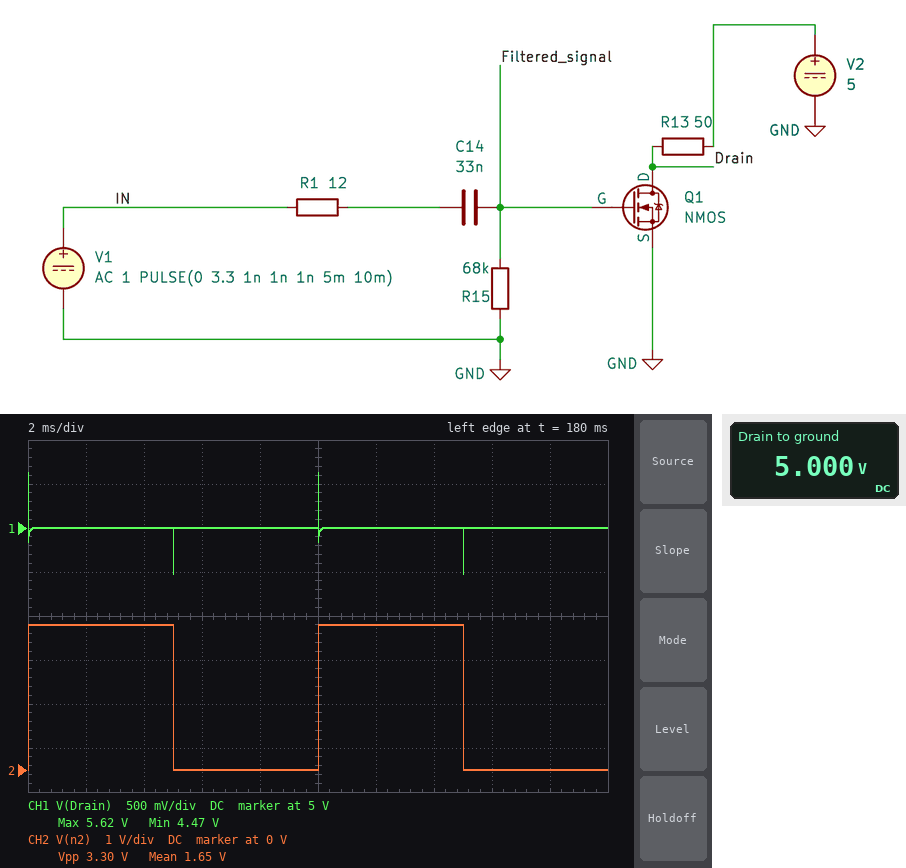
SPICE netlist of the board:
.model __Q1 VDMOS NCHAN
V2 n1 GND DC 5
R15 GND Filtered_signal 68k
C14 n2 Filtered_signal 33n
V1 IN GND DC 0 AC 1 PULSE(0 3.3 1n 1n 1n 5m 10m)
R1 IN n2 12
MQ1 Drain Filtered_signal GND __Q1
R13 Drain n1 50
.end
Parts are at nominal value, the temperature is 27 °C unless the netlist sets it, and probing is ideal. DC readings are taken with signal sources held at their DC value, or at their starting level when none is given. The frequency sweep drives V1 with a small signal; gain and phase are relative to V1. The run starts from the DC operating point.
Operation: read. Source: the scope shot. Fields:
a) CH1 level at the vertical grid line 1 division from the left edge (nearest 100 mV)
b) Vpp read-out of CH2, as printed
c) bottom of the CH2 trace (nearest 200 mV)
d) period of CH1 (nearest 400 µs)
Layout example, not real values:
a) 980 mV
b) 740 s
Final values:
a) 5.0 V
b) 3.30 V
c) 0 V
d) 10.0 ms
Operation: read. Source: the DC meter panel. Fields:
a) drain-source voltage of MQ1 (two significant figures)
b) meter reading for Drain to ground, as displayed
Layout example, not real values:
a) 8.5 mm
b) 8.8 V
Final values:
a) 5.0 V
b) 5.000 V
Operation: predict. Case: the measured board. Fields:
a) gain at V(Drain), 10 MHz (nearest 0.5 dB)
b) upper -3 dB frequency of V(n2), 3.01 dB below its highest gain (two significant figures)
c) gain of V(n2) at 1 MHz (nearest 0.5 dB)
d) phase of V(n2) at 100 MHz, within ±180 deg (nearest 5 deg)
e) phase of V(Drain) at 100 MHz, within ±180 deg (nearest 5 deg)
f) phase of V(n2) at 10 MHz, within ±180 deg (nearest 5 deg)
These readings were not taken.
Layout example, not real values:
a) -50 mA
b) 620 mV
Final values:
a) -13.0 dB
b) 8.8 MHz
c) 0 dB
d) -85 deg
e) -80 deg
f) -45 deg
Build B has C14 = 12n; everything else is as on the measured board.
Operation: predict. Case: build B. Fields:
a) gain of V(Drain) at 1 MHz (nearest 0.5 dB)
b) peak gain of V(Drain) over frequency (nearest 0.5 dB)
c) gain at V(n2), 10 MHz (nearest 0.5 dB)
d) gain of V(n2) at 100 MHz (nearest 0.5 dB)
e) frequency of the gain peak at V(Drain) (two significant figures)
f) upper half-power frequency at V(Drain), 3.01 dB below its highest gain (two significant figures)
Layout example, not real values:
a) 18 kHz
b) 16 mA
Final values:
a) -26.5 dB
b) -13.0 dB
c) -3.0 dB
d) -20.0 dB
e) 9.5 MHz
f) 23 MHz
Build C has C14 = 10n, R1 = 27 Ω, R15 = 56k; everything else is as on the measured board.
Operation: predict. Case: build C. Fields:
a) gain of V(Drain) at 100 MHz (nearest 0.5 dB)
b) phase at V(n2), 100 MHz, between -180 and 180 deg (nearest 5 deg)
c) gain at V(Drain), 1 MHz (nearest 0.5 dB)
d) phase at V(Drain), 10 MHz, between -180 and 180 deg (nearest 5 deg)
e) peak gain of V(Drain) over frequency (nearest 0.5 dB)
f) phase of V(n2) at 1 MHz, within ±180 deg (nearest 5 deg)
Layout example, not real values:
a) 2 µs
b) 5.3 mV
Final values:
a) -34.5 dB
b) -85 deg
c) -27.0 dB
d) -25 deg
e) -17.5 dB
f) -15 deg
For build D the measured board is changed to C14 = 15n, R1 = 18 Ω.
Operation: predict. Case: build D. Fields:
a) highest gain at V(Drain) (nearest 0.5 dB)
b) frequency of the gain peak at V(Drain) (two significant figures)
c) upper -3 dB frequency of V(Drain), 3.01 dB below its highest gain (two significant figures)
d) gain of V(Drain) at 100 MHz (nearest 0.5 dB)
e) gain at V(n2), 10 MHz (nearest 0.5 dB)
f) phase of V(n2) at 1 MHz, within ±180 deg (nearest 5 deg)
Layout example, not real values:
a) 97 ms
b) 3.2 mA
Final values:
a) -15.0 dB
b) 7.6 MHz
c) 19 MHz
d) -31.0 dB
e) -5.5 dB
f) -10 deg
